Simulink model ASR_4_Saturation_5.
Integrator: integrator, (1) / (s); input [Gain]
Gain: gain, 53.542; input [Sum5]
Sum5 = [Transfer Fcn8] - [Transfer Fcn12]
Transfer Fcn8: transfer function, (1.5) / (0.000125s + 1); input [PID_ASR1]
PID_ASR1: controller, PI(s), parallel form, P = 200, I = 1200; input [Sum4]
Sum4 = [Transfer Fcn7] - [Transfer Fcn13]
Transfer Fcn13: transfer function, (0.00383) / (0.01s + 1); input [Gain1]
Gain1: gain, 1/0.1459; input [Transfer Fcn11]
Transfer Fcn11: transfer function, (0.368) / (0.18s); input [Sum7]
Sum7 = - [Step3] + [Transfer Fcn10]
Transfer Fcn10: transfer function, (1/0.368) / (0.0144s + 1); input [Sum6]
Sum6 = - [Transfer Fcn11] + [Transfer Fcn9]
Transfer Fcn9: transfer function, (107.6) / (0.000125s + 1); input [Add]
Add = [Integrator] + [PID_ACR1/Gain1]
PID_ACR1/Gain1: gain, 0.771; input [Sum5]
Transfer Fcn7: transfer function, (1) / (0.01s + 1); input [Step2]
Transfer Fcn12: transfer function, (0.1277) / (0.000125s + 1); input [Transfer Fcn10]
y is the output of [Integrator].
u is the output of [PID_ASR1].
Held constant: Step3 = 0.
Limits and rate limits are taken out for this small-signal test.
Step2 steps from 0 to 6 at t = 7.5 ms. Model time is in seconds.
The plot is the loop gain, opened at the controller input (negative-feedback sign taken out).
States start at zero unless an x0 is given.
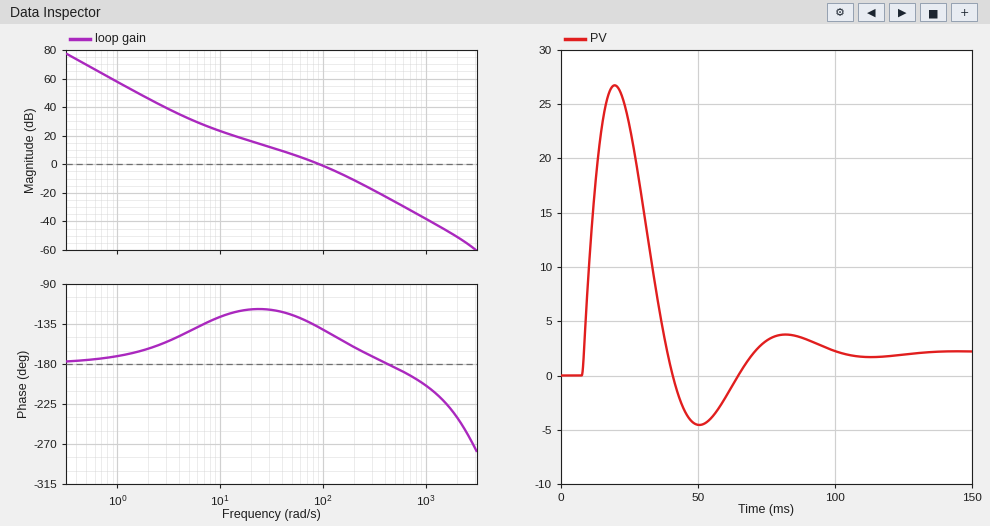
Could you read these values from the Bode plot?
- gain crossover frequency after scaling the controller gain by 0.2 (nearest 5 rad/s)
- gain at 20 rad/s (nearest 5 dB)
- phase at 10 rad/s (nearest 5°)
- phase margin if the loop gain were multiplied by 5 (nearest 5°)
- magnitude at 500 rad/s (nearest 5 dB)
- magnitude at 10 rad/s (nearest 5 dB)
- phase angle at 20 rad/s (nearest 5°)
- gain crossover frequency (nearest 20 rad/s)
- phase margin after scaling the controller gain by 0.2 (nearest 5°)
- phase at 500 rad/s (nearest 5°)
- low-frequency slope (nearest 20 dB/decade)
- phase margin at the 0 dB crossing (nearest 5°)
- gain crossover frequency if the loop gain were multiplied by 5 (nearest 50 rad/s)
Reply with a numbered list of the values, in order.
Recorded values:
1. 25 rad/s
2. 15 dB
3. -125°
4. 15°
5. -25 dB
6. 25 dB
7. -120°
8. 100 rad/s
9. 60°
10. -185°
11. -40 dB/decade
12. 40°
13. 250 rad/s
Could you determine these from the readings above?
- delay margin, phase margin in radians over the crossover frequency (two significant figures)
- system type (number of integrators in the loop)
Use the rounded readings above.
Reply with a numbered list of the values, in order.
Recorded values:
1. 0.0070 s
2. 2
